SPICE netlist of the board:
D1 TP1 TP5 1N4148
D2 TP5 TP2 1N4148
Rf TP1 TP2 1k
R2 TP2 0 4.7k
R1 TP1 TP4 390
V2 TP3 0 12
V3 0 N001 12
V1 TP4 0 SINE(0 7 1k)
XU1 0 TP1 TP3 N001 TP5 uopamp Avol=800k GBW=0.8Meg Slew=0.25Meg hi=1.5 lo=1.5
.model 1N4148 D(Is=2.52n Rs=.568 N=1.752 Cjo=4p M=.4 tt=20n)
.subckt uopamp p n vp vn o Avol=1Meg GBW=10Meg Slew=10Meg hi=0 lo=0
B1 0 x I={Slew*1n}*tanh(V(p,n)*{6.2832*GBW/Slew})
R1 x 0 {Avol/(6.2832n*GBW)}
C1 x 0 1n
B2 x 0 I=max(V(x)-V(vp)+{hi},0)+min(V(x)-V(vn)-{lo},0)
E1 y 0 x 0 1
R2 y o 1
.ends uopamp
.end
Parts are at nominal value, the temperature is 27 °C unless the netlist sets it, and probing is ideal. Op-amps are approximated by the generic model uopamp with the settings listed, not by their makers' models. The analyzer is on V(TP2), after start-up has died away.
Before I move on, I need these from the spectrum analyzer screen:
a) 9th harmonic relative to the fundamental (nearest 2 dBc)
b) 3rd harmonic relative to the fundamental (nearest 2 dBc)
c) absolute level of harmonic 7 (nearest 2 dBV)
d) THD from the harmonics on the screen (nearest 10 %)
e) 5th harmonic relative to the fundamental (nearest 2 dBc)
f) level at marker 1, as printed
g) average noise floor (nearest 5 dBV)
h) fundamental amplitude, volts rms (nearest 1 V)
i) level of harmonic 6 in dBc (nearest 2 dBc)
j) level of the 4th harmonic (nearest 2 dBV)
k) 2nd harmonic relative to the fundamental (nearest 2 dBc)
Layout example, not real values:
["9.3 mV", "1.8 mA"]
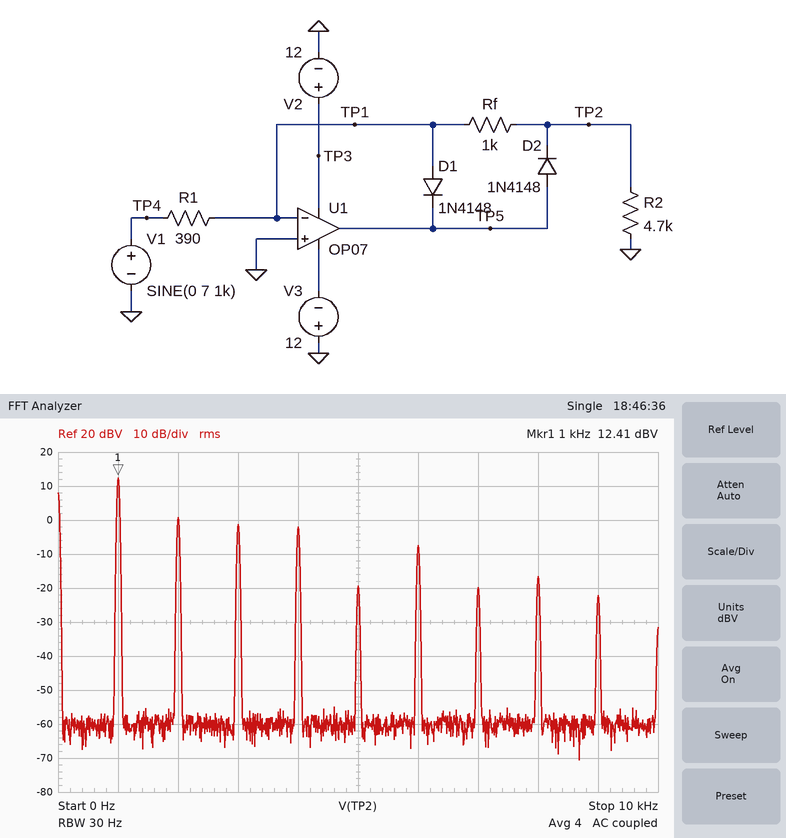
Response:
["-34 dBc", "-14 dBc", "-20 dBV", "40 %", "-32 dBc", "12.41 dBV", "-60 dBV", "4 V", "-20 dBc", "-2 dBV", "-12 dBc"]
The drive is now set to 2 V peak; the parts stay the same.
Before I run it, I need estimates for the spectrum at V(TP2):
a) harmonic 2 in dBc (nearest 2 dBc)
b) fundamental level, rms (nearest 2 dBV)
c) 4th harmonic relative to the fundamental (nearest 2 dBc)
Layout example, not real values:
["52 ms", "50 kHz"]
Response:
["-8 dBc", "6 dBV", "-22 dBc"]
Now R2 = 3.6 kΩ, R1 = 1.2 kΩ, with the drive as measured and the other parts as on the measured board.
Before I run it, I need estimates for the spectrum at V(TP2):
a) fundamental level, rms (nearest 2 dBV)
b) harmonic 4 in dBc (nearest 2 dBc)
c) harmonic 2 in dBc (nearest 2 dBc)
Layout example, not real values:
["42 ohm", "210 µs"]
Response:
["6 dBV", "-22 dBc", "-8 dBc"]
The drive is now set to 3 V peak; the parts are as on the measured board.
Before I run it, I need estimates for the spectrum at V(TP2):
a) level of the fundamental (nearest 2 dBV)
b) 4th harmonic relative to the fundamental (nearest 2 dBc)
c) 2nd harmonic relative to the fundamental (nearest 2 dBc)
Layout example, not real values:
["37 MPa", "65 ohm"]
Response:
["8 dBV", "-22 dBc", "-8 dBc"]
